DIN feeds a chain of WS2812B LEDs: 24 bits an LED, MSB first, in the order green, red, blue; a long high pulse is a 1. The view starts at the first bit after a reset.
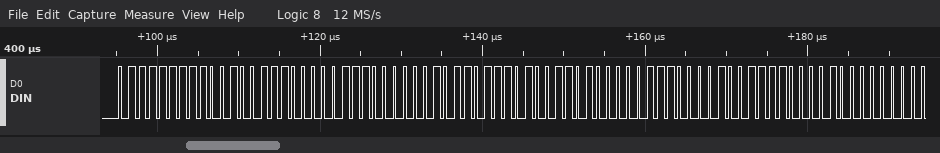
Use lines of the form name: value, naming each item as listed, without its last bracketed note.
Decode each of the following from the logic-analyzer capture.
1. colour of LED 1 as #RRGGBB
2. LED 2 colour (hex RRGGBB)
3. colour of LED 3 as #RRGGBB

colour of LED 1 as #RRGGBB: #937F83
LED 2 colour: #6E819A
colour of LED 3 as #RRGGBB: #130EC2
